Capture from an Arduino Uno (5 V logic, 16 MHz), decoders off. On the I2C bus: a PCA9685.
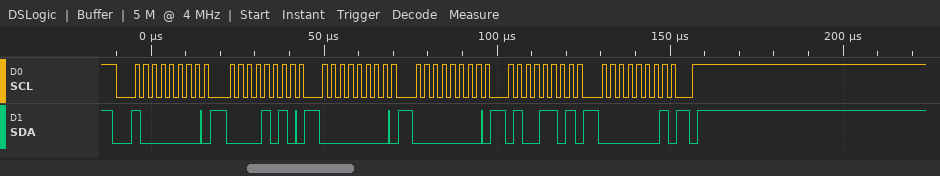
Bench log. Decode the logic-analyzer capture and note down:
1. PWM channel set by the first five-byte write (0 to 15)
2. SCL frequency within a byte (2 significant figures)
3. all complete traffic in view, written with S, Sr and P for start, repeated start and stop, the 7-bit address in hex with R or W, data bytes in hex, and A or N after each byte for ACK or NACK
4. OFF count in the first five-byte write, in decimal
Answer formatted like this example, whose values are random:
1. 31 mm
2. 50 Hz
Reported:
1. 1
2. 400 kHz
3. S 40W A 0A A 00 A 00 A 4D A 01 A P
4. 333
